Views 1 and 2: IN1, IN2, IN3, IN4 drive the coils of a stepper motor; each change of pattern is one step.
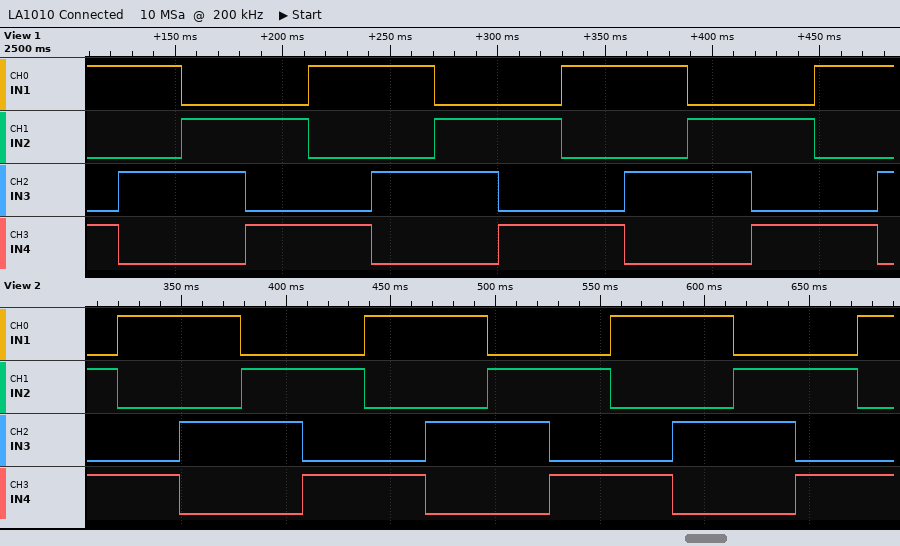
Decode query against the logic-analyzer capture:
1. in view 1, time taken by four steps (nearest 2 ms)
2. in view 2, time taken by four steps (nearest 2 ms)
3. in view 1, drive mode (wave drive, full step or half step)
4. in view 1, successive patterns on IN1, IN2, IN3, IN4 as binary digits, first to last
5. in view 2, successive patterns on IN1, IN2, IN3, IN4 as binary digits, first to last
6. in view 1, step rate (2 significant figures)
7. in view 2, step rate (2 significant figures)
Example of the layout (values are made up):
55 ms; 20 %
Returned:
118 ms; 118 ms; full step; 1001 1010 0110 0101 1001 1010 0110 0101 1001 1010 0110 0101 1001 1010; 0101 1001 1010 0110 0101 1001 1010 0110 0101 1001 1010 0110 0101 1001; 34 steps/s; 34 steps/s
